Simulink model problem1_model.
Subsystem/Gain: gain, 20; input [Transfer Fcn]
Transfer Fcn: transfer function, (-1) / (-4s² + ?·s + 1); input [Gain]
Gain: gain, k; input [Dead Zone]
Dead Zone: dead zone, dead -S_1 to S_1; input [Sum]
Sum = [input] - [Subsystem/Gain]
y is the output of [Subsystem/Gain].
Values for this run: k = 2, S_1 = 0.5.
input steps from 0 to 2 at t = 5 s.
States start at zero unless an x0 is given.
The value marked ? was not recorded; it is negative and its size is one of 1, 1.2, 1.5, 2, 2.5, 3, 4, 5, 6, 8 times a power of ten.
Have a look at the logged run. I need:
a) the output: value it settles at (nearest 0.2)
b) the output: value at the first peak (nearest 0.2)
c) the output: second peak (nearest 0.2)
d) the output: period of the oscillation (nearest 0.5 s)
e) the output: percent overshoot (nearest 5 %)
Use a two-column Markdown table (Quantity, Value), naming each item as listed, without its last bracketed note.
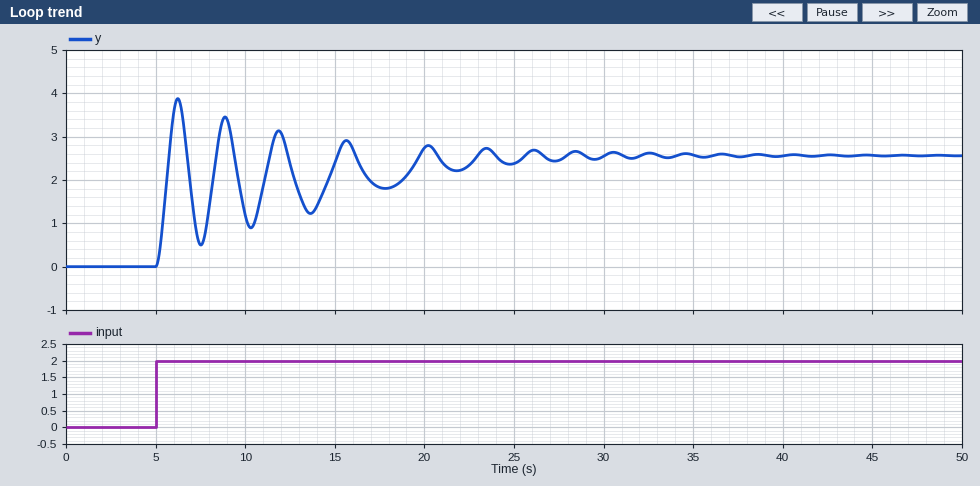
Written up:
| Quantity | Value |
|---|---|
| the output: value it settles at | 2.6 |
| the output: value at the first peak | 3.8 |
| the output: second peak | 3.4 |
| the output: period of the oscillation | 2.5 s |
| the output: percent overshoot | 50 % |
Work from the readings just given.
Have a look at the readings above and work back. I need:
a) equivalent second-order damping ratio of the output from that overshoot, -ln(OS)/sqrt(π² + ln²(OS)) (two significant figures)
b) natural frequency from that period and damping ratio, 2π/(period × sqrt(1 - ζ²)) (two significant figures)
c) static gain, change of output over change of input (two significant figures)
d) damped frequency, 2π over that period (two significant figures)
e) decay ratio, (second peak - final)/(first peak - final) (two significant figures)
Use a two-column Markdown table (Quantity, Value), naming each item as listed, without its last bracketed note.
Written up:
| Quantity | Value |
|---|---|
| equivalent second-order damping ratio of the output from that overshoot, -ln(OS)/sqrt(π² + ln²(OS)) | 0.22 |
| natural frequency from that period and damping ratio, 2π/(period × sqrt(1 - ζ²)) | 2.6 rad/s |
| static gain, change of output over change of input | 1.3 |
| damped frequency, 2π over that period | 2.5 rad/s |
| decay ratio, (second peak - final)/(first peak - final) | 0.67 |
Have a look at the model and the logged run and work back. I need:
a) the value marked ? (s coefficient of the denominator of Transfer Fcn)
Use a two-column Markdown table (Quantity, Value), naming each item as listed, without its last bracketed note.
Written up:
| Quantity | Value |
|---|---|
| the value marked ? | -1 |
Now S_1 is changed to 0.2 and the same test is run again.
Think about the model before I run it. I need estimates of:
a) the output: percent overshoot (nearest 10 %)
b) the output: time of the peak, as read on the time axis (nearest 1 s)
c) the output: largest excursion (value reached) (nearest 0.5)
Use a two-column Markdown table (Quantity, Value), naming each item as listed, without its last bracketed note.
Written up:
| Quantity | Value |
|---|---|
| the output: percent overshoot | 70 % |
| the output: time of the peak, as read on the time axis | 6 s |
| the output: largest excursion (value reached) | 4.0 |
